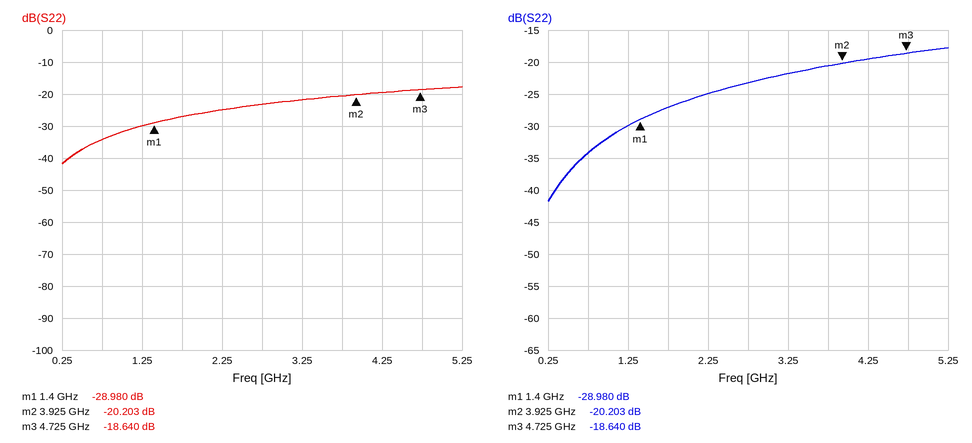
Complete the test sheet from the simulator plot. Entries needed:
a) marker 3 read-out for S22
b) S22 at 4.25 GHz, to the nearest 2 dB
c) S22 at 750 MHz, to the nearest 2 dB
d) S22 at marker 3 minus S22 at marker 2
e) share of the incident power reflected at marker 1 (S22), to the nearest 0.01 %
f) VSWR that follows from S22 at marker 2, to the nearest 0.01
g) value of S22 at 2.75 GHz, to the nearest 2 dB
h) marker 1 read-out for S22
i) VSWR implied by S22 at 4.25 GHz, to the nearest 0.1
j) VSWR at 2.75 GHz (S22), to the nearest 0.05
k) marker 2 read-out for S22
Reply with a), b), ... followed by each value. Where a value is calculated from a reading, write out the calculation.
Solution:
a) -18.640 dB
b) -20 dB
c) -34 dB
d) -18.64 − (-20.203) = 1.563 dB
e) 10^(-28.98/10) ≈ 0.13 %
f) (1 + 0.0977)/(1 − 0.0977) ≈ 1.22
g) -24 dB
h) -28.980 dB
i) |Γ| = 10^(-20/20) = 0.1000; VSWR = (1 + 0.1000)/(1 − 0.1000) ≈ 1.2
j) |Γ| = 10^(-24/20) = 0.0631; VSWR = (1 + 0.0631)/(1 − 0.0631) ≈ 1.13, so 1.15 to the nearest 0.05
k) -20.203 dB
